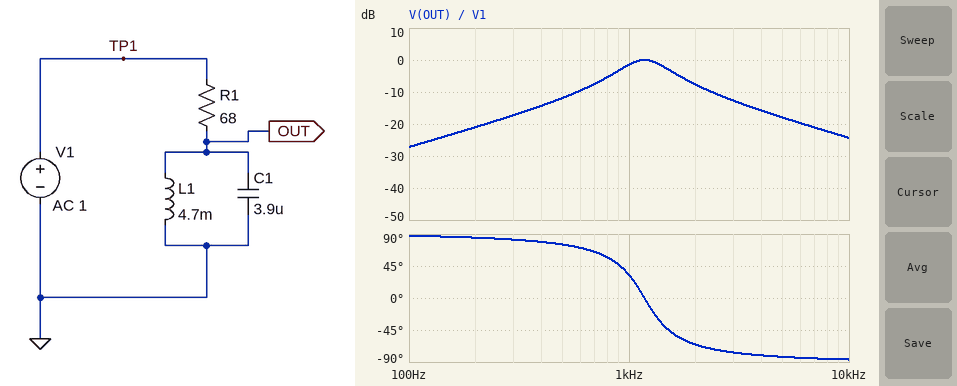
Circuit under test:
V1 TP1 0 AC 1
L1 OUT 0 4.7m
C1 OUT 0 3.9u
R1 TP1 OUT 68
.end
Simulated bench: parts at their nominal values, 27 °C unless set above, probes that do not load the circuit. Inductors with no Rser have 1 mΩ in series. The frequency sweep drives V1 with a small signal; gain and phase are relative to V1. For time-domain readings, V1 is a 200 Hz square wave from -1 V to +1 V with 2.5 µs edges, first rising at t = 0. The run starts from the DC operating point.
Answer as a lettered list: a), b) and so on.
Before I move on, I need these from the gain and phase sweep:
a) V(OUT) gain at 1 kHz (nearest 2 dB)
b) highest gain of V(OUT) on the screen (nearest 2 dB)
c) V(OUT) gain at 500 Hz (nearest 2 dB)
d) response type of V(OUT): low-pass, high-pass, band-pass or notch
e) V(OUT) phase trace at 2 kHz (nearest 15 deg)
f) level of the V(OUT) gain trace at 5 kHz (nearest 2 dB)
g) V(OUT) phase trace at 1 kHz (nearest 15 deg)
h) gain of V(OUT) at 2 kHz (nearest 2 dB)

a) -2 dB
b) 0 dB
c) -12 dB
d) band-pass
e) -60 deg
f) -18 dB
g) 30 deg
h) -8 dB
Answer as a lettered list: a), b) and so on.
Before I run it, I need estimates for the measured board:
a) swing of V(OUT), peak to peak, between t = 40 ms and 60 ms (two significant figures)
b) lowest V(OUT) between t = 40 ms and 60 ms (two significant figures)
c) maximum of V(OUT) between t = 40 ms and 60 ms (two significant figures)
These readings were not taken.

a) 1.4 V
b) -720 mV
c) 720 mV
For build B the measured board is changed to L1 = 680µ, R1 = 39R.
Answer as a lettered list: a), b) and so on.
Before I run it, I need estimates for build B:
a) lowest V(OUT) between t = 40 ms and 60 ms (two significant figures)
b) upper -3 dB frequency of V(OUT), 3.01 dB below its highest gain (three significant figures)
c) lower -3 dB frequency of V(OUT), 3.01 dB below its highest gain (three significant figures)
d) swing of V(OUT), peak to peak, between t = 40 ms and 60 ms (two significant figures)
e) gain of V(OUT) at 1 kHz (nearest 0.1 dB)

a) -530 mV
b) 3.66 kHz
c) 2.61 kHz
d) 1.1 V
e) -18.3 dB
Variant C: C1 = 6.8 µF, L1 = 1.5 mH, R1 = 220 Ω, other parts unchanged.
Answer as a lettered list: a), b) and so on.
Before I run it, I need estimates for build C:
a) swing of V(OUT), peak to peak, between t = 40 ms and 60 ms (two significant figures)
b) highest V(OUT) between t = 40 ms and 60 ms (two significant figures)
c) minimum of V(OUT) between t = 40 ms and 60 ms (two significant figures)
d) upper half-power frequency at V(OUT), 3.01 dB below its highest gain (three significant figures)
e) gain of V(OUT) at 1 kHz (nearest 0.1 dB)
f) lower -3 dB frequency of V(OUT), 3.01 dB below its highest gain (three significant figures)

a) 180 mV
b) 92 mV
c) -92 mV
d) 1.63 kHz
e) -22.9 dB
f) 1.52 kHz
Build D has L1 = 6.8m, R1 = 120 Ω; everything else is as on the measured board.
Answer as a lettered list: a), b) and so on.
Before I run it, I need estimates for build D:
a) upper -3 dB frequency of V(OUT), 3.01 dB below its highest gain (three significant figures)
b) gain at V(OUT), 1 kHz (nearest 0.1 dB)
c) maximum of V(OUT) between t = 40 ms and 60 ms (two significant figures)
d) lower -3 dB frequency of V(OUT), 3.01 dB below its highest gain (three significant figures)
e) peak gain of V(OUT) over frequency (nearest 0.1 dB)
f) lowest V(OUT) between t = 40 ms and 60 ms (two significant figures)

a) 1.16 kHz
b) -0.1 dB
c) 570 mV
d) 822 Hz
e) 0 dB
f) -570 mV
